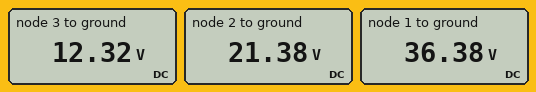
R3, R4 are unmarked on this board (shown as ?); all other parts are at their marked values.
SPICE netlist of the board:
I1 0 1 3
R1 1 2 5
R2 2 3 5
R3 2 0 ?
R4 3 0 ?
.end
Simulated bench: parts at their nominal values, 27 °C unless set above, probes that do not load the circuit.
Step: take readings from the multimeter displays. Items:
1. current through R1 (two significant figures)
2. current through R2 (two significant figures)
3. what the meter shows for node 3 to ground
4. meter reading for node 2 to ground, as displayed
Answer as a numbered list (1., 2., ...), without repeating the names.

1. 3.0 A
2. 1.8 A
3. 12.32 V
4. 21.38 V
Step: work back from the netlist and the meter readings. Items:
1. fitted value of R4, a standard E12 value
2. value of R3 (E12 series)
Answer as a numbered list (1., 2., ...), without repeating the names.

1. 6.8 Ω
2. 18 Ω
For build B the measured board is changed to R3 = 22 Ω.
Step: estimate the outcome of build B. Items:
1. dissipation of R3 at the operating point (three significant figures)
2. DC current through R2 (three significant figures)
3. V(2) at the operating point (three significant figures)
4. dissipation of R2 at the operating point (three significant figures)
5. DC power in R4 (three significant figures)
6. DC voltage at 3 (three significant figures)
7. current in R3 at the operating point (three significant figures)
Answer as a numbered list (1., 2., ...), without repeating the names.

1. 24.1 W
2. 1.95 A
3. 23.0 V
4. 19.1 W
5. 25.9 W
6. 13.3 V
7. 1.05 A
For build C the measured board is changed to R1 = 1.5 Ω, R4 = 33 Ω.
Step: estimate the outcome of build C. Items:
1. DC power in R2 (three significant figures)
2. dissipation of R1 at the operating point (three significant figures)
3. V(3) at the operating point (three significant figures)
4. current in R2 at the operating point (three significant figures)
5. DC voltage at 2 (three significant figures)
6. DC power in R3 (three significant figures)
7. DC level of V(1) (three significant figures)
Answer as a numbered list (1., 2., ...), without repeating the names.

1. 4.65 W
2. 13.5 W
3. 31.8 V
4. 964 mA
5. 36.6 V
6. 74.6 W
7. 41.1 V
